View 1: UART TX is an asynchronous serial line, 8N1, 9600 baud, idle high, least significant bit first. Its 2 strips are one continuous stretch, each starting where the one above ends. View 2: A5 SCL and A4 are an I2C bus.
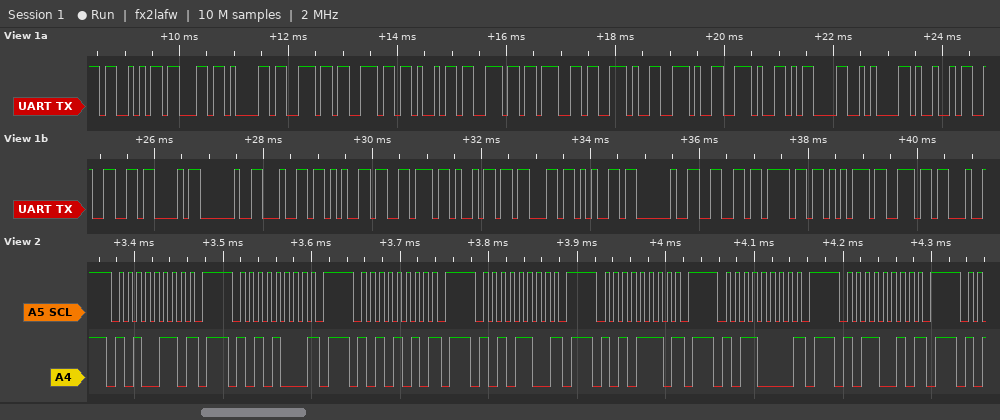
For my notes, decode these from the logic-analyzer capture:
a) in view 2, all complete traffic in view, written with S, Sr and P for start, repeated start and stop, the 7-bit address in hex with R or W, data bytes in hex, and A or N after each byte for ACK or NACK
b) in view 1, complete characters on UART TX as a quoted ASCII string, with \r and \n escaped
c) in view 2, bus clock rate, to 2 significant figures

S 53W N P S 54W N P S 55W N P S 56W N P S 57W N P S 58W N P S 59W N P
"Scanning...\r\nI2C device foun"
100 kHz
